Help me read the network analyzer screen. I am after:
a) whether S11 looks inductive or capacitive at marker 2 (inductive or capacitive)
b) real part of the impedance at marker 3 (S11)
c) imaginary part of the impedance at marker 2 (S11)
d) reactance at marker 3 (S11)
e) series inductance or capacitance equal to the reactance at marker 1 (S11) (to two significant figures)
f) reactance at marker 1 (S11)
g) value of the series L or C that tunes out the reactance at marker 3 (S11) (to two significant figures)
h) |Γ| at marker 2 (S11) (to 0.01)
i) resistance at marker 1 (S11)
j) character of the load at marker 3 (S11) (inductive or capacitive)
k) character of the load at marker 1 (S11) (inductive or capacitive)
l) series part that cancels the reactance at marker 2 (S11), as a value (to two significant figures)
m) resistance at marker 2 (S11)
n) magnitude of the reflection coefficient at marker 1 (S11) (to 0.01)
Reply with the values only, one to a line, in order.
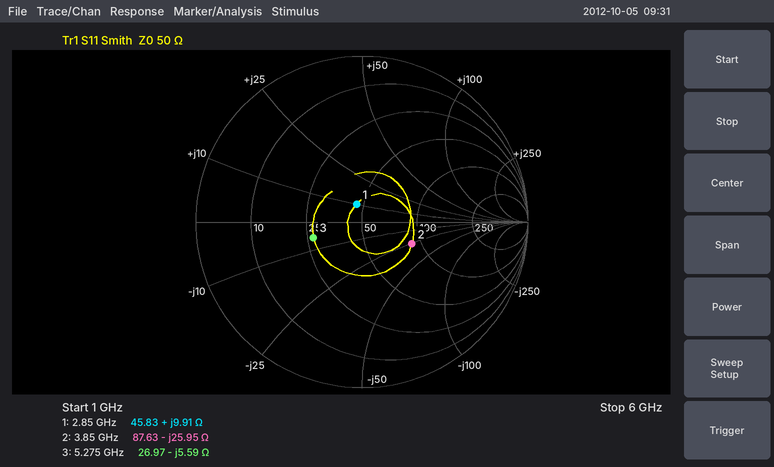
capacitive
26.97 Ω
-25.95 Ω
-5.59 Ω
550 pH
+9.91 Ω
170 pH
0.33
45.83 Ω
capacitive
inductive
1.1 nH
87.63 Ω
0.11
